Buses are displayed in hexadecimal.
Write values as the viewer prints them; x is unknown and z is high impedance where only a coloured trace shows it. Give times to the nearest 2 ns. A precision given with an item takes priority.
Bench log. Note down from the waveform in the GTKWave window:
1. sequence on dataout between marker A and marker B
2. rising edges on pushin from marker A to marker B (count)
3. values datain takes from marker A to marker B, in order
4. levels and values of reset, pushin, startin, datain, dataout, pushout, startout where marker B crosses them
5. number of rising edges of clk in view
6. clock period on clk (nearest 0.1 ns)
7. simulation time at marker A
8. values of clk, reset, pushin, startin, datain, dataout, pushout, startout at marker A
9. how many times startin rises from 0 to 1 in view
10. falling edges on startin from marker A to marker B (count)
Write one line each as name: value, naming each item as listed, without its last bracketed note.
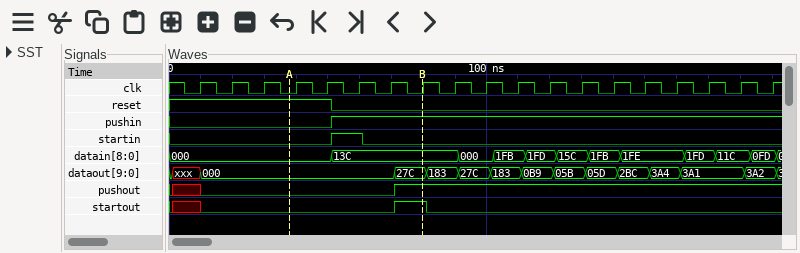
sequence on dataout between marker A and marker B: 000, 27C
rising edges on pushin from marker A to marker B: 1
values datain takes from marker A to marker B, in order: 000, 13C
levels and values of reset, pushin, startin, datain, dataout, pushout, startout where marker B crosses them: reset=0, pushin=1, startin=0, datain=13C, dataout=27C, pushout=1, startout=1
number of rising edges of clk in view: 19
clock period on clk: 10 ns
simulation time at marker A: 38 ns
values of clk, reset, pushin, startin, datain, dataout, pushout, startout at marker A: clk=0, reset=1, pushin=0, startin=0, datain=000, dataout=000, pushout=0, startout=0
how many times startin rises from 0 to 1 in view: 1
falling edges on startin from marker A to marker B: 1
